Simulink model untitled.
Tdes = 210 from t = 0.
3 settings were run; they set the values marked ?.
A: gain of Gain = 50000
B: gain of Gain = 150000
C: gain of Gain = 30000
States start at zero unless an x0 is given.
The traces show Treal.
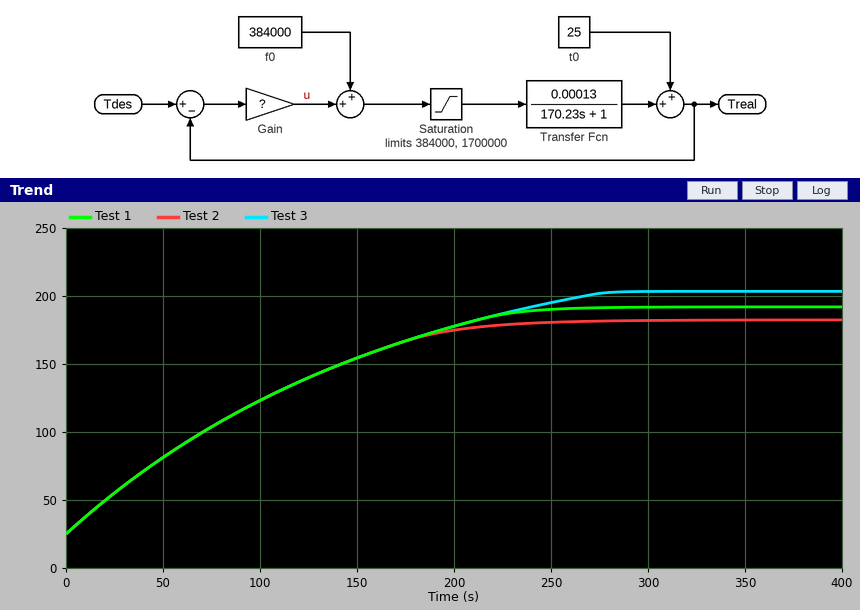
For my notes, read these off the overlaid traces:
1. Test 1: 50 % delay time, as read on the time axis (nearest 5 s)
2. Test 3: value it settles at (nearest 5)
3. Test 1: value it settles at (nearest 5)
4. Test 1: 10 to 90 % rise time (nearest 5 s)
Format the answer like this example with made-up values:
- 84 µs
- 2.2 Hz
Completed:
- 80 s
- 205
- 190
- 180 s
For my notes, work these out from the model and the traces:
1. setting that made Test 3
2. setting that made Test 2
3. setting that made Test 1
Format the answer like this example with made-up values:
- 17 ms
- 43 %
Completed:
- B
- C
- A
